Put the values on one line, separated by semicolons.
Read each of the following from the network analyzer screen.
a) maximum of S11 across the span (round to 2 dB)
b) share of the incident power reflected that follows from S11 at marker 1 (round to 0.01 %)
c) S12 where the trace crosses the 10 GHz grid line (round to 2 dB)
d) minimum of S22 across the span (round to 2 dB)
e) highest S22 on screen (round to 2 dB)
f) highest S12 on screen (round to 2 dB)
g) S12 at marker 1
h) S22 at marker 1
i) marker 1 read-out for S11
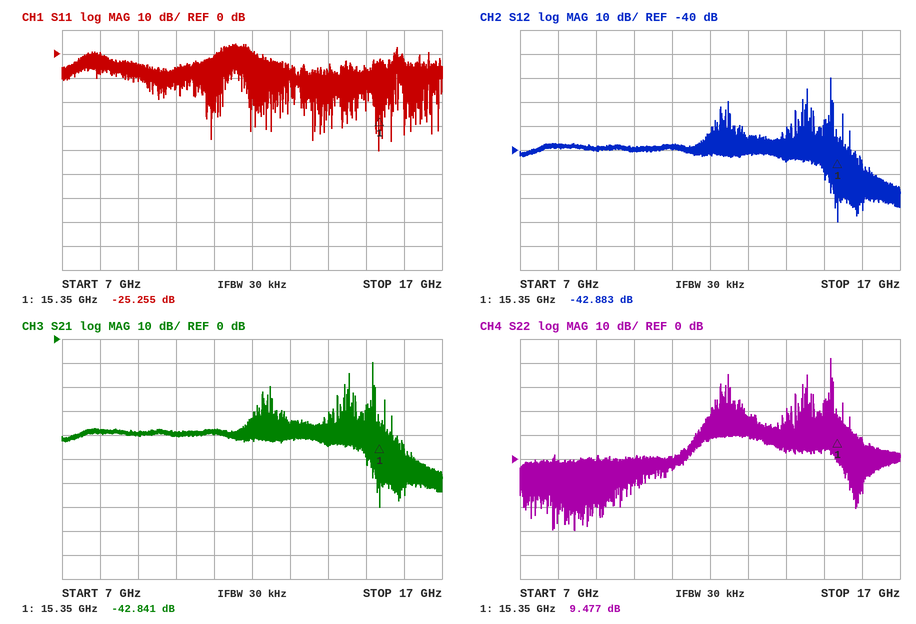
4 dB; 0.30 %; -40 dB; -30 dB; 42 dB; -10 dB; -42.883 dB; 9.477 dB; -25.255 dB
